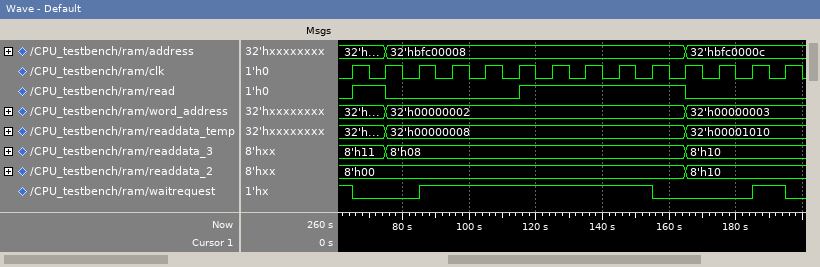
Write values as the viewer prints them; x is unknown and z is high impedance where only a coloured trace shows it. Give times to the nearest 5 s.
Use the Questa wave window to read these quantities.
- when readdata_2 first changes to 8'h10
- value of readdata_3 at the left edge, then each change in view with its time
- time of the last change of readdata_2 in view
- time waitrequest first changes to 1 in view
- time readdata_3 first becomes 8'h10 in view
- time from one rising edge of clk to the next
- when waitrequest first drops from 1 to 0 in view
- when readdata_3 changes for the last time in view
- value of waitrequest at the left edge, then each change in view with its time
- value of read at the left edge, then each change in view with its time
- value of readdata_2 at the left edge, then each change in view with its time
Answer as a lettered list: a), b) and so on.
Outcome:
a) 165 s
b) 8'h11, 8'h08 at 75 s, 8'h10 at 165 s
c) 165 s
d) 85 s
e) 165 s
f) 10 s
g) 65 s
h) 165 s
i) 1, 0 at 65 s, 1 at 85 s, 0 at 155 s, 1 at 185 s, 0 at 195 s
j) 0, 1 at 65 s, 0 at 75 s, 1 at 115 s, 0 at 165 s
k) 8'h00, 8'h10 at 165 s
